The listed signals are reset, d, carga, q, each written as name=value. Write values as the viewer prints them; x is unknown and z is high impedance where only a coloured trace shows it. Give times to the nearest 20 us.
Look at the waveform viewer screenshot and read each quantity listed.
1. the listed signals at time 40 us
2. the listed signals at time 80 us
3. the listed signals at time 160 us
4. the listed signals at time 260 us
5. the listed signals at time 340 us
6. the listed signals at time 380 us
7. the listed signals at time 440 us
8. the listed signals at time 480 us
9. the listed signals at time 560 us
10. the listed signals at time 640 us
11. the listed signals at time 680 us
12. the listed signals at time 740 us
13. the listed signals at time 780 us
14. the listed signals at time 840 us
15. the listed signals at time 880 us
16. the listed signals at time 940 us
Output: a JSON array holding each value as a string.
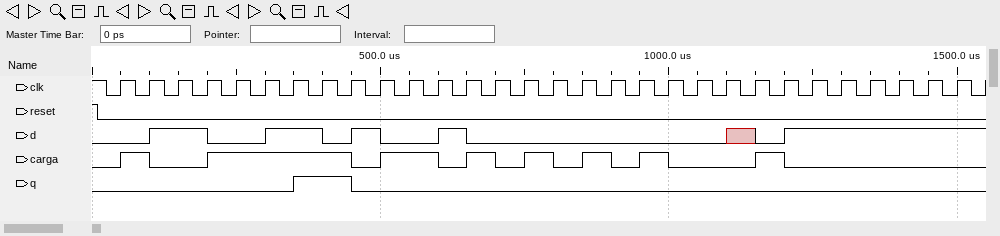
["reset=0, d=0, carga=0, q=0", "reset=0, d=0, carga=1, q=0", "reset=0, d=1, carga=0, q=0", "reset=0, d=0, carga=1, q=0", "reset=0, d=1, carga=1, q=0", "reset=0, d=1, carga=1, q=1", "reset=0, d=0, carga=1, q=1", "reset=0, d=1, carga=0, q=0", "reset=0, d=0, carga=1, q=0", "reset=0, d=1, carga=0, q=0", "reset=0, d=0, carga=1, q=0", "reset=0, d=0, carga=0, q=0", "reset=0, d=0, carga=1, q=0", "reset=0, d=0, carga=0, q=0", "reset=0, d=0, carga=1, q=0", "reset=0, d=0, carga=0, q=0"]
